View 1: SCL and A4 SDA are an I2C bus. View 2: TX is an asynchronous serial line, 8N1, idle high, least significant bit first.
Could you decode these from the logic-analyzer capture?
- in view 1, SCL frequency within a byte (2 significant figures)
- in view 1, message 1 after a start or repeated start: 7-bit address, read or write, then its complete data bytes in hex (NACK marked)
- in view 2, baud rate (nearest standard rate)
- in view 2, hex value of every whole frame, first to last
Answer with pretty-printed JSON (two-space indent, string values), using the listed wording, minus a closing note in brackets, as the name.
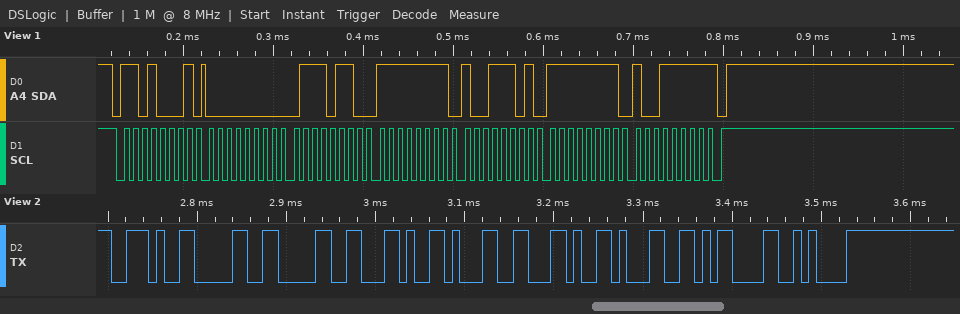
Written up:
{
  "in view 1, SCL frequency within a byte": "100 kHz",
  "in view 1, message 1 after a start or repeated start: 7-bit address, read or write, then its complete data bytes in hex": "0x68 read: 00 76 FF 9D FF 9F NACK",
  "in view 2, baud rate": "115200 baud",
  "in view 2, hex value of every whole frame, first to last": "2E 30 30 2C 31 2C 31 0D 0A"
}
